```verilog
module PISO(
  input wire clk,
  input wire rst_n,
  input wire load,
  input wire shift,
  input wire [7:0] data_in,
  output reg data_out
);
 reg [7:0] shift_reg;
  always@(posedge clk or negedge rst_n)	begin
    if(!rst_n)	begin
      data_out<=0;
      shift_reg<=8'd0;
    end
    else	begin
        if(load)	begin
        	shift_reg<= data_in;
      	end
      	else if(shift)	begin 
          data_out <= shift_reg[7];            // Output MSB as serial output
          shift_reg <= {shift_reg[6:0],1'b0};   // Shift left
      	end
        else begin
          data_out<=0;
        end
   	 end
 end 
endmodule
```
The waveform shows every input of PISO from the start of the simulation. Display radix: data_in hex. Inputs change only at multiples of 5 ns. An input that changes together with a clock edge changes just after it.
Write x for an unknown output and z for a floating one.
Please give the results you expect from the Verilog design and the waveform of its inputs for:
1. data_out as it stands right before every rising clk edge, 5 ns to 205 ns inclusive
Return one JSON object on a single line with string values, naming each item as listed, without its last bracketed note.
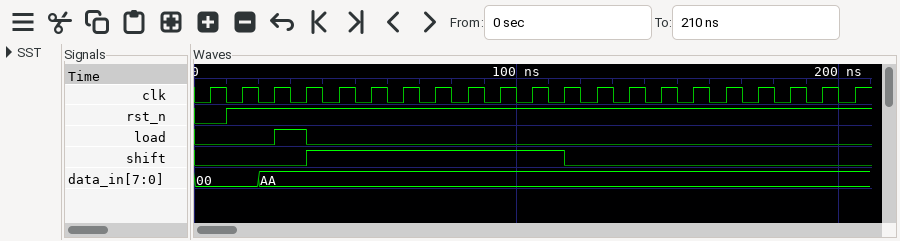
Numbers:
{"data_out as it stands right before every rising clk edge, 5 ns to 205 ns inclusive": "0 0 0 0 0 1 0 1 0 1 0 1 0 0 0 0 0 0 0 0 0"}
